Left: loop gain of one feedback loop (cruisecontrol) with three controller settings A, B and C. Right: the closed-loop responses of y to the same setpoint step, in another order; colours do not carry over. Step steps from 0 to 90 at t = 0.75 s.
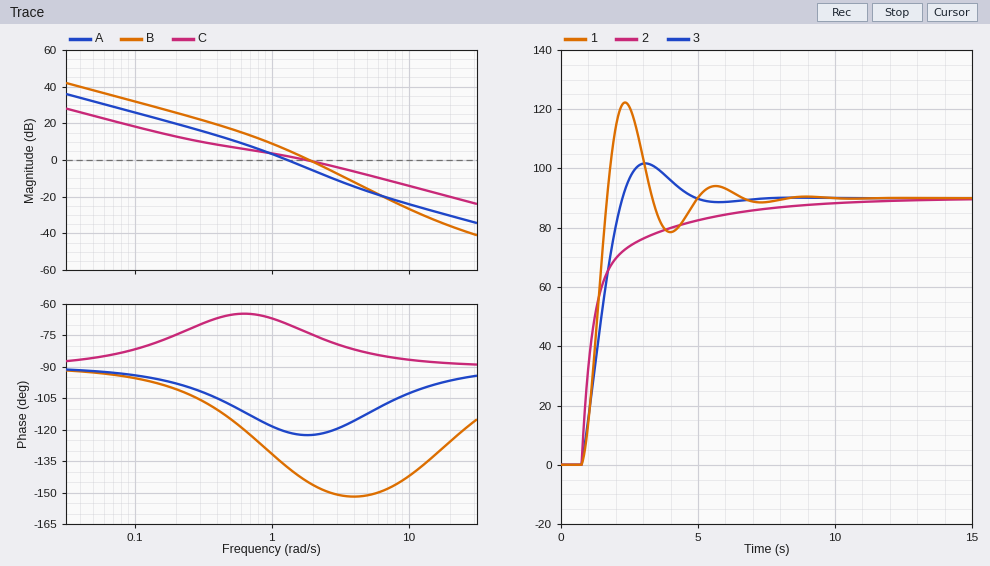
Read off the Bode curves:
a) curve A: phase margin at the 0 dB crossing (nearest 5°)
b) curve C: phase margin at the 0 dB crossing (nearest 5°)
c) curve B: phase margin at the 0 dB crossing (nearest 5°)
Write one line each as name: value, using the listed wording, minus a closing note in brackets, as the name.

curve A: phase margin at the 0 dB crossing: 60°
curve C: phase margin at the 0 dB crossing: 105°
curve B: phase margin at the 0 dB crossing: 35°
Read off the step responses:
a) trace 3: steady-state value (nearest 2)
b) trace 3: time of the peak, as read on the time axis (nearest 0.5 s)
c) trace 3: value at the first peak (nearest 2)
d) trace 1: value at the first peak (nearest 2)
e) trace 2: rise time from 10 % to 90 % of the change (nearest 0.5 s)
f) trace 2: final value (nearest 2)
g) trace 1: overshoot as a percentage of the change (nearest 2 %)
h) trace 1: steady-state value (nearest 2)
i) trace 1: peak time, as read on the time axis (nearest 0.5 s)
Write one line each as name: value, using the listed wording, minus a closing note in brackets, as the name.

trace 3: steady-state value: 90
trace 3: time of the peak, as read on the time axis: 3.0 s
trace 3: value at the first peak: 102
trace 1: value at the first peak: 122
trace 2: rise time from 10 % to 90 % of the change: 3.5 s
trace 2: final value: 90
trace 1: overshoot as a percentage of the change: 36 %
trace 1: steady-state value: 90
trace 1: peak time, as read on the time axis: 2.5 s
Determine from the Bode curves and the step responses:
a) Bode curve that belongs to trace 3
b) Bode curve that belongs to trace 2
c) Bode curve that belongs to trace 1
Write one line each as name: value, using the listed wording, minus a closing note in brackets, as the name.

Bode curve that belongs to trace 3: A
Bode curve that belongs to trace 2: C
Bode curve that belongs to trace 1: B
